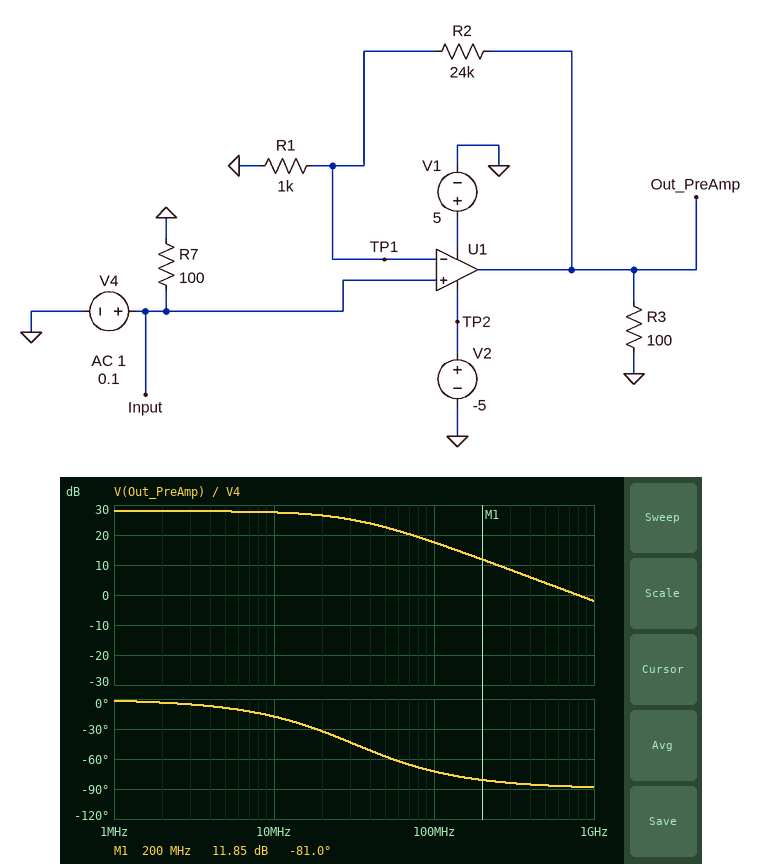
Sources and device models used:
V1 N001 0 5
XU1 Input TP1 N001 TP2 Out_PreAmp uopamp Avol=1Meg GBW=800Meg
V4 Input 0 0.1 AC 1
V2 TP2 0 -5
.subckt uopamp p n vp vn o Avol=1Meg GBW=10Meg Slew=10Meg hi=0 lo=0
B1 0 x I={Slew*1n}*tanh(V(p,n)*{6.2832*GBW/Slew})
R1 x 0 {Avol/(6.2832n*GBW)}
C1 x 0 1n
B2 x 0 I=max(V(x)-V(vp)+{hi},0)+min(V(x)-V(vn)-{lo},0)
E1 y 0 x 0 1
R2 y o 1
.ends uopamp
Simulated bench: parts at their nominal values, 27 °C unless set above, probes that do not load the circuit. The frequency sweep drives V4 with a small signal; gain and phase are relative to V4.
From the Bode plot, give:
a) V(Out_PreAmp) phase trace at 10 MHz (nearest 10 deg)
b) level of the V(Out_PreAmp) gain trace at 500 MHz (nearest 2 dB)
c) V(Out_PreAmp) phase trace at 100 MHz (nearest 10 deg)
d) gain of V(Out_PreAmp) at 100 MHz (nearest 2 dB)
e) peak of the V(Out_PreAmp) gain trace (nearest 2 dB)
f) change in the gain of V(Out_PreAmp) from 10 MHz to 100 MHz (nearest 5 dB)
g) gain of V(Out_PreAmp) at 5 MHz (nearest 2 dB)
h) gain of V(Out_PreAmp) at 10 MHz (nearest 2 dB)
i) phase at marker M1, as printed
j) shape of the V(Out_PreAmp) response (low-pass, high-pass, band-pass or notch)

-20 deg
4 dB
-70 deg
18 dB
28 dB
-10 dB
28 dB
28 dB
-81.0 deg
low-pass
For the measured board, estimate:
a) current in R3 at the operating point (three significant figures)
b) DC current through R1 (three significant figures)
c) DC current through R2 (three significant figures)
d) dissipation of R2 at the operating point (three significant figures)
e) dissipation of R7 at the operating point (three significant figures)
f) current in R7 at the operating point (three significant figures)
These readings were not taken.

25.0 mA
100 µA
100 µA
240 µW
100 µW
1.00 mA
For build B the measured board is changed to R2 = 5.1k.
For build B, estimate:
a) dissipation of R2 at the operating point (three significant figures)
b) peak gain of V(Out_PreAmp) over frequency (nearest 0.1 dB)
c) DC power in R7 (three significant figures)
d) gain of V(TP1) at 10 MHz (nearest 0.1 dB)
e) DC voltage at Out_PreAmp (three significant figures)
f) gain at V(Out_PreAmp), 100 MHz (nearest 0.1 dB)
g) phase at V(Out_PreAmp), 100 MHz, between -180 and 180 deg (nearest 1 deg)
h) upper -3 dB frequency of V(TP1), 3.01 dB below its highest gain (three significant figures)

51.0 µW
15.7 dB
100 µW
0 dB
610 mV
13.7 dB
-38 deg
130 MHz
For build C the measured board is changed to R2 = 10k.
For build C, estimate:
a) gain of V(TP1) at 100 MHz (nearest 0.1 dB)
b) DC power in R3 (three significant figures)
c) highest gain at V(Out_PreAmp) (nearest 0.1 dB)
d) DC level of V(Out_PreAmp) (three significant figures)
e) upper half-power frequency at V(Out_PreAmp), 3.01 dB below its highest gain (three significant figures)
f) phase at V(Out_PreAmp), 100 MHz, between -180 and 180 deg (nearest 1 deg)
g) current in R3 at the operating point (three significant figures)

-4.7 dB
12.1 mW
20.8 dB
1.10 V
72.0 MHz
-54 deg
11.0 mA
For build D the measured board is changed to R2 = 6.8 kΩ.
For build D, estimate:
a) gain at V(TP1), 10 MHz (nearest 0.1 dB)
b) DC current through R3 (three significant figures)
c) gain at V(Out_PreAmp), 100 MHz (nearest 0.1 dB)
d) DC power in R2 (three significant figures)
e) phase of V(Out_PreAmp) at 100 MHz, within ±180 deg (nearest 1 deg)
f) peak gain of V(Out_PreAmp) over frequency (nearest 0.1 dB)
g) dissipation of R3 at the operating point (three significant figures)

0 dB
7.80 mA
14.9 dB
68.0 µW
-45 deg
17.8 dB
6.08 mW
